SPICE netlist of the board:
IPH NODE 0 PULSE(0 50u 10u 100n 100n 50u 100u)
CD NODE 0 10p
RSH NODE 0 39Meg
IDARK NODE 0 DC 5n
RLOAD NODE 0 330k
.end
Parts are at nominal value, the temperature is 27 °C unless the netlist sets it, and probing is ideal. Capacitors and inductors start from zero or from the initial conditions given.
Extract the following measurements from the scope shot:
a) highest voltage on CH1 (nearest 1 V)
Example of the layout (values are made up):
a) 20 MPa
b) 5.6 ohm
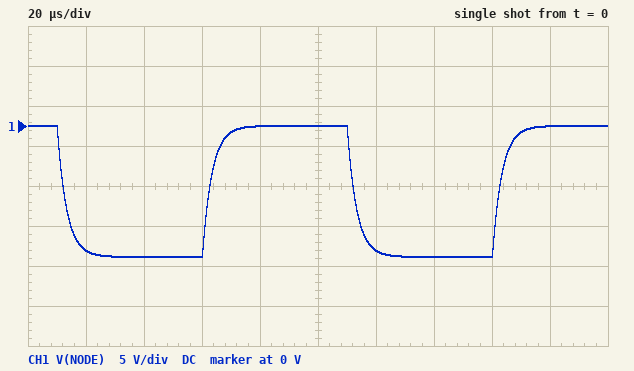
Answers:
a) 0 V
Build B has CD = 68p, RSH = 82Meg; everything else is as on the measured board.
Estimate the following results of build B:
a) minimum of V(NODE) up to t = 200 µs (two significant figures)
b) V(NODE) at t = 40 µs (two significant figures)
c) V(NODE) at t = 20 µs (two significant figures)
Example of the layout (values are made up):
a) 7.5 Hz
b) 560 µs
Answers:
a) -15 V
b) -12 V
c) -5.9 V
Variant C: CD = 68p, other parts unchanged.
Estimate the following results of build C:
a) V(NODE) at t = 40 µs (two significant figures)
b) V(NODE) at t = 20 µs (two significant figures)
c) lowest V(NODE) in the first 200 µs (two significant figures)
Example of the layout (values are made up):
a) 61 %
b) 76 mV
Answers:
a) -12 V
b) -5.9 V
c) -15 V
